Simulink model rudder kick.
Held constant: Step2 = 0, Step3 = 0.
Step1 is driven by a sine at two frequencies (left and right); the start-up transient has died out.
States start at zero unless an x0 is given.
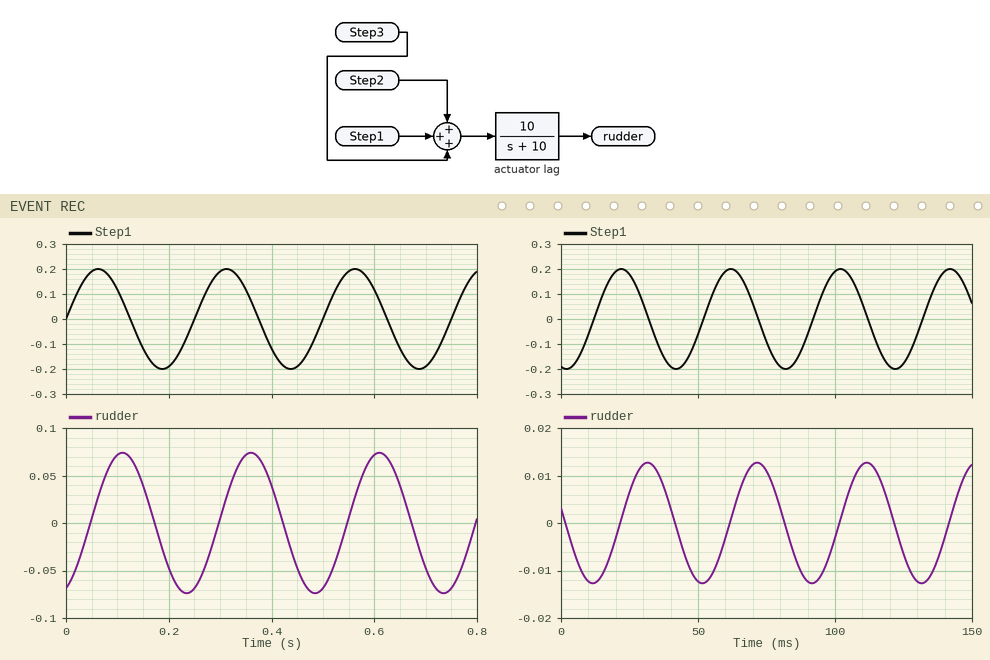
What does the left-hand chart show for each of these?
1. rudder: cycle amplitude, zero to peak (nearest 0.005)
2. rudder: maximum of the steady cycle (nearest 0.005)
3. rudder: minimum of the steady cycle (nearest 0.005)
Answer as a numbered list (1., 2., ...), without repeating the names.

1. 0.075
2. 0.075
3. -0.075
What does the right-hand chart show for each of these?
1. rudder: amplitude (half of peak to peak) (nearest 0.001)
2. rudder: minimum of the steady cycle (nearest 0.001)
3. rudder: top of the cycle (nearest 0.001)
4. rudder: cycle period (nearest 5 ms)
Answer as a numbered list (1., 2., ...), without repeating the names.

1. 0.013
2. -0.013
3. 0.013
4. 40 ms
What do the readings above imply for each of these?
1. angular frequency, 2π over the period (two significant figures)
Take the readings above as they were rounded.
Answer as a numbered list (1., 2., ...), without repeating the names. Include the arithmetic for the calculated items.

1. 2π / 40 = 0.16 rad/ms
